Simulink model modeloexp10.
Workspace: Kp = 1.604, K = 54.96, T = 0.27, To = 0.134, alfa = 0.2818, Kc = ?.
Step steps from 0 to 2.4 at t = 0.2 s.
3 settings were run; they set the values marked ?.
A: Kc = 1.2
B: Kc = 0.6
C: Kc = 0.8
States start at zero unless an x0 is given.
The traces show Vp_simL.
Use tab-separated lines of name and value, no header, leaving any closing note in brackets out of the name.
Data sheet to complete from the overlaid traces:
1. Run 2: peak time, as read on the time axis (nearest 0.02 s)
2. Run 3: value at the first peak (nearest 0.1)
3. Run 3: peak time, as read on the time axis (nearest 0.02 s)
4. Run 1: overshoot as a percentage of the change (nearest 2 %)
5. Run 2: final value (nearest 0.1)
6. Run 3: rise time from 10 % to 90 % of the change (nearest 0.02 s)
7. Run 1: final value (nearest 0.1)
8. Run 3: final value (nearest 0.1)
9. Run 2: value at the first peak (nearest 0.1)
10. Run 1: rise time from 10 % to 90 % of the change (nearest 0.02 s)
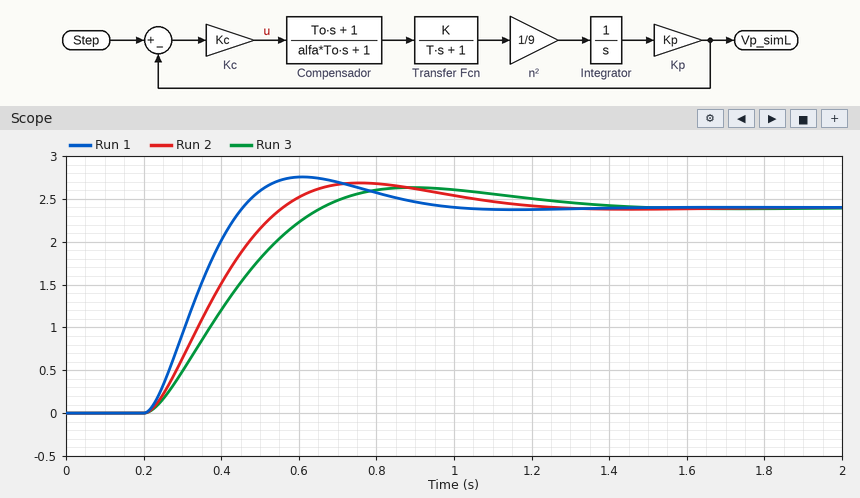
Run 2: peak time, as read on the time axis	0.76 s
Run 3: value at the first peak	2.6
Run 3: peak time, as read on the time axis	0.90 s
Run 1: overshoot as a percentage of the change	14 %
Run 2: final value	2.4
Run 3: rise time from 10 % to 90 % of the change	0.32 s
Run 1: final value	2.4
Run 3: final value	2.4
Run 2: value at the first peak	2.7
Run 1: rise time from 10 % to 90 % of the change	0.18 s
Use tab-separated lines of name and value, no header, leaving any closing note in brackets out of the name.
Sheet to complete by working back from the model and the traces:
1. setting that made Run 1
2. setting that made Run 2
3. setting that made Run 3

setting that made Run 1	A
setting that made Run 2	C
setting that made Run 3	B
